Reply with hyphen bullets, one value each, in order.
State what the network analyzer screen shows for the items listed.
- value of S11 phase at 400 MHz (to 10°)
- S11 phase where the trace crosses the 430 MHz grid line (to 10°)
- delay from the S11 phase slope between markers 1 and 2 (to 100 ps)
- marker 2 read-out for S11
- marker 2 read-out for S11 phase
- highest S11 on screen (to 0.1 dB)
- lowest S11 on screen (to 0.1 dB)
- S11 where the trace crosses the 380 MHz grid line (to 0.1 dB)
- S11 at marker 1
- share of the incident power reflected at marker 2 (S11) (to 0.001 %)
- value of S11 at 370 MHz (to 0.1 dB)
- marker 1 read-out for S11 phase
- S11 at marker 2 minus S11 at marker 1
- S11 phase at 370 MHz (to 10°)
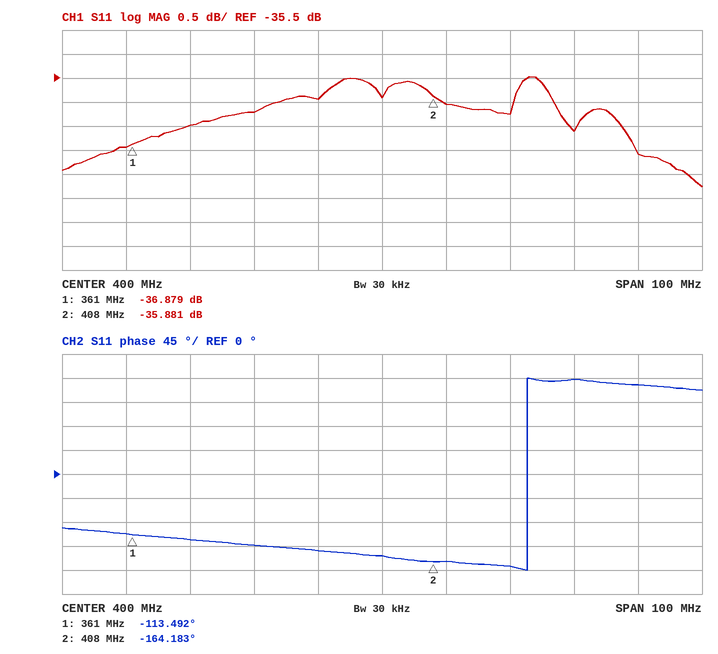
- -150°
- 180°
- 3.0 ns
- -35.881 dB
- -164.183°
- -35.5 dB
- -37.8 dB
- -36.2 dB
- -36.879 dB
- 0.026 %
- -36.5 dB
- -113.492°
- 0.998 dB
- -120°
